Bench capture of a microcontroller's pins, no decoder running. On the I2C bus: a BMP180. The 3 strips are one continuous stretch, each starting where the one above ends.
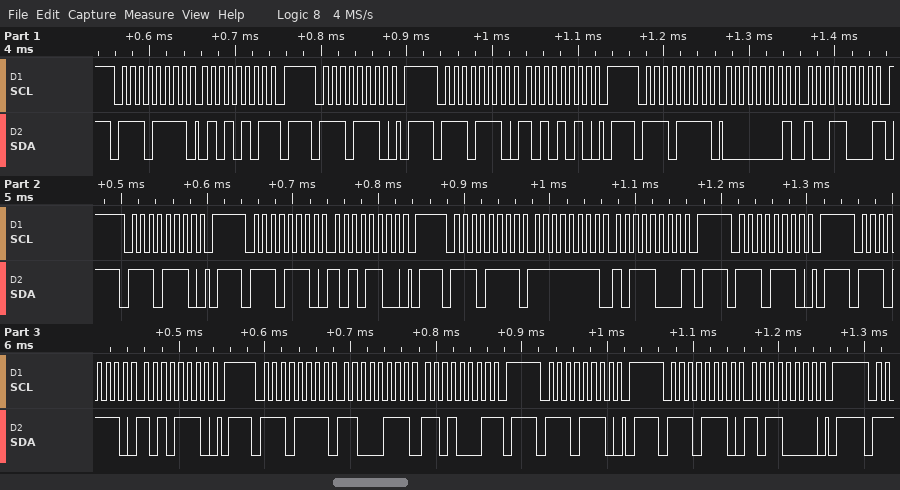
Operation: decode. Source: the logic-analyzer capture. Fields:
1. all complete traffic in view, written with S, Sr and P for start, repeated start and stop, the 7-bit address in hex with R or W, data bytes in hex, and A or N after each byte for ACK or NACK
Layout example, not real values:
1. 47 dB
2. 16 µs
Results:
1. S 77R A 55 N P S 77W A P S 77W A AA A P S 77R A 01 A 98 N P S 77W A P S 77W A AC A P S 77R A FF A B8 N P S 77W A P S 77W A AE A P S 77R A C7 A D1 N P S 77W A P S 77W A B0 A P
